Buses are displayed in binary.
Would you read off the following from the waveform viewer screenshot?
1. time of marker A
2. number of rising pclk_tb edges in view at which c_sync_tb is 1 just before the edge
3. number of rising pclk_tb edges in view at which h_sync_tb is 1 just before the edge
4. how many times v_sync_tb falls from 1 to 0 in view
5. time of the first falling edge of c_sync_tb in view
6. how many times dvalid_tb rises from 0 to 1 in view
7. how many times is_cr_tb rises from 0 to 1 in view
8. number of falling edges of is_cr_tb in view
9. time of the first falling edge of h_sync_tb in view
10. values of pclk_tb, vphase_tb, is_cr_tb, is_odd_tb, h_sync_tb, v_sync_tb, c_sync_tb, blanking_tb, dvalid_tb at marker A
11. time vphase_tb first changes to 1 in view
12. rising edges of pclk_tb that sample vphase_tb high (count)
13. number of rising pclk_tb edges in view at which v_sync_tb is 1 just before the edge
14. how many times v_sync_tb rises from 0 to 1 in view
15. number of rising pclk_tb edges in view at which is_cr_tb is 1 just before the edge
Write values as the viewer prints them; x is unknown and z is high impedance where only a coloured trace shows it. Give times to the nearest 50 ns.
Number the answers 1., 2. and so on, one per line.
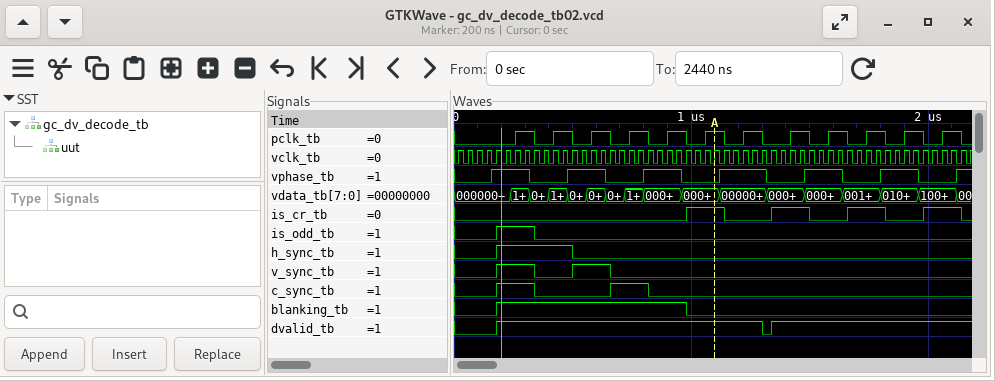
1. 1100 ns
2. 2
3. 2
4. 2
5. 350 ns
6. 2
7. 4
8. 4
9. 500 ns
10. pclk_tb=1, vphase_tb=0, is_cr_tb=1, is_odd_tb=0, h_sync_tb=0, v_sync_tb=0, c_sync_tb=0, blanking_tb=0, dvalid_tb=1
11. 150 ns
12. 6
13. 2
14. 2
15. 4
